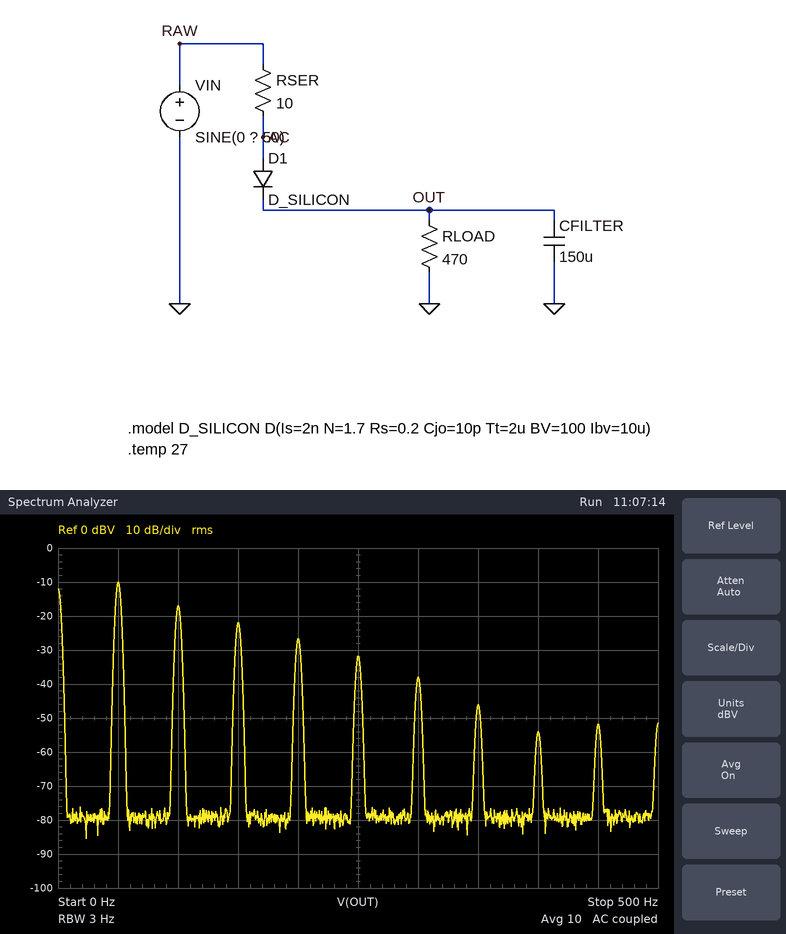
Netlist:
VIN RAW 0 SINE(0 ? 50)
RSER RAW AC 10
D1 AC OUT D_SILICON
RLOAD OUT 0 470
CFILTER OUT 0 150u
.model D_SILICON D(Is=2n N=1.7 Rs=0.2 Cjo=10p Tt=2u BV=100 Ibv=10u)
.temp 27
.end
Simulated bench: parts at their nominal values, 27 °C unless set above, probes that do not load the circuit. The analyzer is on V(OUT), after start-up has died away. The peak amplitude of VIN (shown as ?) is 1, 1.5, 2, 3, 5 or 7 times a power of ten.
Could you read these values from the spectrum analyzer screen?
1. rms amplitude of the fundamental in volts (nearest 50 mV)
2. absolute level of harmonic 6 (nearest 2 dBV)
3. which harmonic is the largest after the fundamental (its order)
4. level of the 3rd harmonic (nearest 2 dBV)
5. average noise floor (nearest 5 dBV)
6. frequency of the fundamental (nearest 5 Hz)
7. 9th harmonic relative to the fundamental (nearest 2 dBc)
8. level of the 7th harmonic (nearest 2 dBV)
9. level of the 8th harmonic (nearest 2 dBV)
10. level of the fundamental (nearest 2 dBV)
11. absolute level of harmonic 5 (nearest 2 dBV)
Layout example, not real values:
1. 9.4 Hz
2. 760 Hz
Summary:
1. 300 mV
2. -38 dBV
3. 2
4. -22 dBV
5. -80 dBV
6. 50 Hz
7. -42 dBc
8. -46 dBV
9. -54 dBV
10. -10 dBV
11. -32 dBV
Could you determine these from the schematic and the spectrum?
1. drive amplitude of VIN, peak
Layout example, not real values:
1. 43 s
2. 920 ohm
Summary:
1. 7 V
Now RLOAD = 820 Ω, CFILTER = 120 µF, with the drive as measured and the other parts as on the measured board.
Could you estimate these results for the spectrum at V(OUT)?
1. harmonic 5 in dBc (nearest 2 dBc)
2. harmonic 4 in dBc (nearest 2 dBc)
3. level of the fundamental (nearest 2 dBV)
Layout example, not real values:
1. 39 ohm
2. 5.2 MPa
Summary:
1. -20 dBc
2. -16 dBc
3. -12 dBV
